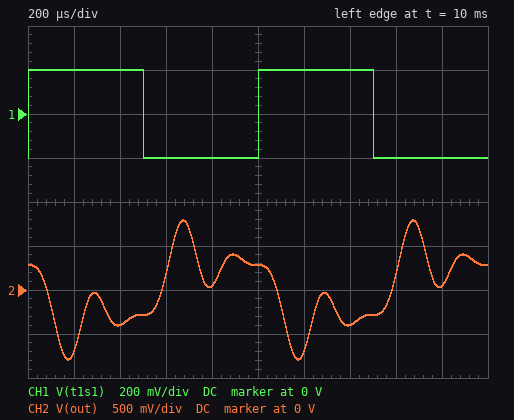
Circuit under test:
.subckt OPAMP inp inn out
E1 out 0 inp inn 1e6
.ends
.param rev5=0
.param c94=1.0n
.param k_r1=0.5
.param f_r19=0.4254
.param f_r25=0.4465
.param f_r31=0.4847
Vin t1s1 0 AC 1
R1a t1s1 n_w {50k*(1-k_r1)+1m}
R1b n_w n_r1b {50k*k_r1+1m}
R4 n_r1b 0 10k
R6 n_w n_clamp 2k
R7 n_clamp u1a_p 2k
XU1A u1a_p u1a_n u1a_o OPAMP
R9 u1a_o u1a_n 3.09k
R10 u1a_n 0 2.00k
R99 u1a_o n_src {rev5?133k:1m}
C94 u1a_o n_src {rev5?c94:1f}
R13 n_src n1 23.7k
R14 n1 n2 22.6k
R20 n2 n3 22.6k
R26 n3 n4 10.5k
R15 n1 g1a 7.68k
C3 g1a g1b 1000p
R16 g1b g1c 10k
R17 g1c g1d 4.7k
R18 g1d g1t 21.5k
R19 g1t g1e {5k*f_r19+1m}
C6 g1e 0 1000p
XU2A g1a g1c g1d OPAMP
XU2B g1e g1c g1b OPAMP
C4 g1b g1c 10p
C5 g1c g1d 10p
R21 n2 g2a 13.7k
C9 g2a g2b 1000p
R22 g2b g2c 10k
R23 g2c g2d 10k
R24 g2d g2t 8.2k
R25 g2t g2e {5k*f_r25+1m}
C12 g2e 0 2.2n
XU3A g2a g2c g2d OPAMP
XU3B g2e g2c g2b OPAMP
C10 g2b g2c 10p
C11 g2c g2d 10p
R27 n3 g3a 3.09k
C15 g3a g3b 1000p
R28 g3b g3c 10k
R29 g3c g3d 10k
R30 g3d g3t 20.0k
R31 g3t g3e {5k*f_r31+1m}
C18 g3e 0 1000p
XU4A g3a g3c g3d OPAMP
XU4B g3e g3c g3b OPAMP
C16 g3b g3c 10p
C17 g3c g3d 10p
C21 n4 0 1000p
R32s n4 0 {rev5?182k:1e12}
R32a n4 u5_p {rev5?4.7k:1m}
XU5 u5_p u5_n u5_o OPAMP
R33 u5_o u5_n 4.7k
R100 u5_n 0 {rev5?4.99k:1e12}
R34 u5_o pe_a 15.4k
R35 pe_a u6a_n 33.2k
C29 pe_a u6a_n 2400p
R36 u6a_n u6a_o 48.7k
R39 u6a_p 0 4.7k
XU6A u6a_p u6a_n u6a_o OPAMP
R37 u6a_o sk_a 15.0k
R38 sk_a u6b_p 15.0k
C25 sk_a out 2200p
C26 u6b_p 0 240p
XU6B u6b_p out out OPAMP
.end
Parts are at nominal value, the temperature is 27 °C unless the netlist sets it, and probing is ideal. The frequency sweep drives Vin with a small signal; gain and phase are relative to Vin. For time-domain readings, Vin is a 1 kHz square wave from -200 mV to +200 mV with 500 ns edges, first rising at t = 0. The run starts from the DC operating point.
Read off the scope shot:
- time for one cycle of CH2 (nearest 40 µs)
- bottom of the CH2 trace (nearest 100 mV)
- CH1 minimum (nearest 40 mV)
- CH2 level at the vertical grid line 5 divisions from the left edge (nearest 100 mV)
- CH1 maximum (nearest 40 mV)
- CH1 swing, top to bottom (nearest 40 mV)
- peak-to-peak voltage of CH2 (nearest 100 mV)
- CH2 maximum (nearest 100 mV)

1.00 ms
-800 mV
-200 mV
300 mV
200 mV
400 mV
1.6 V
800 mV
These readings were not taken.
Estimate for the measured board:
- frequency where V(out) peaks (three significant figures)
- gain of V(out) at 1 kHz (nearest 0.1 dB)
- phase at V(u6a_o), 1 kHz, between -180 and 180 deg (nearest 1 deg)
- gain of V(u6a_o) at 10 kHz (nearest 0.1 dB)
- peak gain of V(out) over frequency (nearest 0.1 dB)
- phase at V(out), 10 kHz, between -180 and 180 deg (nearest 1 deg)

4.03 kHz
4.6 dB
169 deg
-34.4 dB
13.0 dB
-14 deg
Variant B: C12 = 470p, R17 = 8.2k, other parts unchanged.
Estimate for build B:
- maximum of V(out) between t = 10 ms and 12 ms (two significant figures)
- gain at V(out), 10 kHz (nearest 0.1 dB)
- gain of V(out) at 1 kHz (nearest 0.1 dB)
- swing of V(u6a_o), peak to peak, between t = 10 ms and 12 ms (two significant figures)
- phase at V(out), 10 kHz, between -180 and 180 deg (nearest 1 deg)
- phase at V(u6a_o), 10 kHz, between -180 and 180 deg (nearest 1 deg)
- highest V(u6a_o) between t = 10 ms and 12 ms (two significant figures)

700 mV
-21.5 dB
4.1 dB
1.3 V
157 deg
-163 deg
660 mV
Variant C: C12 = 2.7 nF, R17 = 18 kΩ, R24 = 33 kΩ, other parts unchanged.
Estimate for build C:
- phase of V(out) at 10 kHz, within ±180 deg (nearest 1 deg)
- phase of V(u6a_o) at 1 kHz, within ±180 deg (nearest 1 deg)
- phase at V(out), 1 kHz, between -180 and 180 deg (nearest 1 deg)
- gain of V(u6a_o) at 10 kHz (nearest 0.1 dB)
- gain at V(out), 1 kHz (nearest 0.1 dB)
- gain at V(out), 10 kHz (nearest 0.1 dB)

165 deg
166 deg
164 deg
7.1 dB
5.5 dB
10.3 dB
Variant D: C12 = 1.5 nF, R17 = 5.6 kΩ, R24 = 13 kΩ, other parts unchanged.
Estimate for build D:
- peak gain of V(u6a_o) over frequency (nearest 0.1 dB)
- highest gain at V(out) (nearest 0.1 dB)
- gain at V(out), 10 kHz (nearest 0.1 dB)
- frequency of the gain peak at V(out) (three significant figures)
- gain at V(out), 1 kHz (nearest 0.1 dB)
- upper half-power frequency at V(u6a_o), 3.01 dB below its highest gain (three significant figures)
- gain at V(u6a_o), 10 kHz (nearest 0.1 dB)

11.9 dB
12.5 dB
-34.8 dB
4.37 kHz
4.5 dB
6.15 kHz
-37.9 dB
